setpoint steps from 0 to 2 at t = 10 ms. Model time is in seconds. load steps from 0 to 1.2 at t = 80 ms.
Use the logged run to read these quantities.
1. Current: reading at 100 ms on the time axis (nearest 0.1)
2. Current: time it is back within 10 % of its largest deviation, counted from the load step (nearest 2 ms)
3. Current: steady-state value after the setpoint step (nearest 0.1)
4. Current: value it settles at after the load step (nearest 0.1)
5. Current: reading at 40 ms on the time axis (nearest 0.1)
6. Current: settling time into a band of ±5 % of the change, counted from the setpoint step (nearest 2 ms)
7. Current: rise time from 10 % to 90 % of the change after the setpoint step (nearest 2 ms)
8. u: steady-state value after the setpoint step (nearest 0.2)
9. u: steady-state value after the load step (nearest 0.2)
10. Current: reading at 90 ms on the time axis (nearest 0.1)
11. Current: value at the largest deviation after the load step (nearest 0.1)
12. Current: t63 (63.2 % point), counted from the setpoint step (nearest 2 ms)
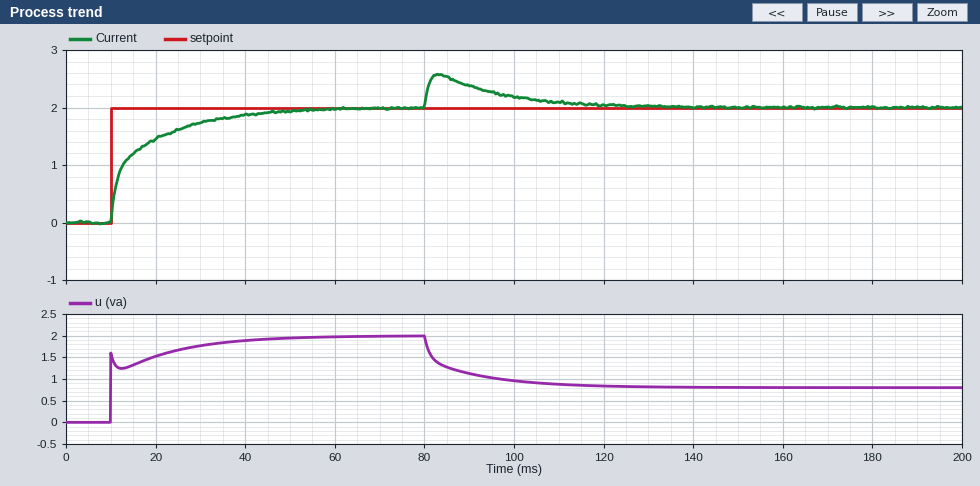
2.2
36 ms
2.0
2.0
1.9
34 ms
24 ms
2.0
0.8
2.4
2.6
6 ms
